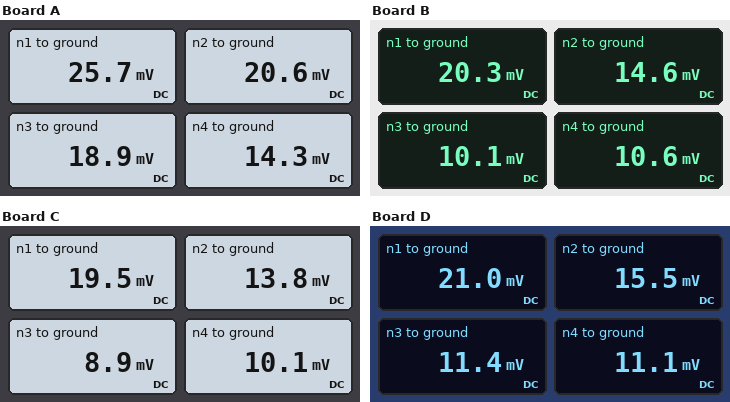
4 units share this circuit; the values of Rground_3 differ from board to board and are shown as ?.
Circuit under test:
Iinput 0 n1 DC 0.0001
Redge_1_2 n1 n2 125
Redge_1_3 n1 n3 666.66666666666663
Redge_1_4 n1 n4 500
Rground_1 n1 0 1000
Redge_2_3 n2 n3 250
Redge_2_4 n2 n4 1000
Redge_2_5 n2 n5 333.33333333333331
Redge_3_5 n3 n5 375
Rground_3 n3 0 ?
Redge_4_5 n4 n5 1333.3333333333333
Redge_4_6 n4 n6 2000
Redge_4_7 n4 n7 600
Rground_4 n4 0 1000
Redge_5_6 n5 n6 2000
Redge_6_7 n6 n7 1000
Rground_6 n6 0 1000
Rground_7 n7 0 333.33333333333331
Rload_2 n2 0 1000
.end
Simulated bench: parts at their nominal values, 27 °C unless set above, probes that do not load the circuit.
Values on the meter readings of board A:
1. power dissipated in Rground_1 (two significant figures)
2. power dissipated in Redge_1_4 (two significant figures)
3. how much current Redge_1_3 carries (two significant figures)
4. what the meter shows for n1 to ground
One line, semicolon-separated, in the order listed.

660 nW; 260 nW; 10 µA; 25.7 mV
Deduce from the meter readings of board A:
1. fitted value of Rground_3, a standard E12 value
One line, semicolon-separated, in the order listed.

1.2 kΩ
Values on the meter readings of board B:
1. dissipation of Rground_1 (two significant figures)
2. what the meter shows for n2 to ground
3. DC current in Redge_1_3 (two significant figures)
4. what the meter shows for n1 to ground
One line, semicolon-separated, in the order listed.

410 nW; 14.6 mV; 15 µA; 20.3 mV
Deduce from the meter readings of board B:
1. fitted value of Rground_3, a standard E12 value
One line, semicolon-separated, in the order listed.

270 Ω
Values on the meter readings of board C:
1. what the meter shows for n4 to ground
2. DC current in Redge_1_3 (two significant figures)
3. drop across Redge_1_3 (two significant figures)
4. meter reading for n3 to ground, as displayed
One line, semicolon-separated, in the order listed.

10.1 mV; 16 µA; 11 mV; 8.9 mV
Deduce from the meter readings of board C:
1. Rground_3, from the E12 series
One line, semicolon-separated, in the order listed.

220 Ω
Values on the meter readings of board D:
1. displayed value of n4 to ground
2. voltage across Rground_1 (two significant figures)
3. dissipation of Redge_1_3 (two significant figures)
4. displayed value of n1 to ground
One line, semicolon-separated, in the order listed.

11.1 mV; 21 mV; 140 nW; 21.0 mV
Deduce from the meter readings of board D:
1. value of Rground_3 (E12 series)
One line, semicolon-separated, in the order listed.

330 Ω
